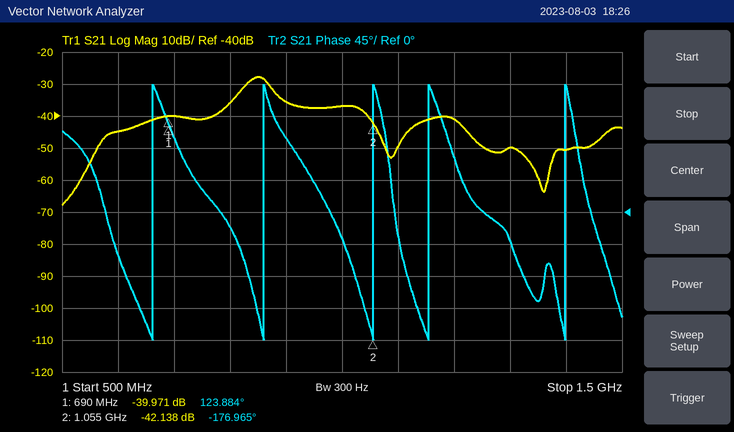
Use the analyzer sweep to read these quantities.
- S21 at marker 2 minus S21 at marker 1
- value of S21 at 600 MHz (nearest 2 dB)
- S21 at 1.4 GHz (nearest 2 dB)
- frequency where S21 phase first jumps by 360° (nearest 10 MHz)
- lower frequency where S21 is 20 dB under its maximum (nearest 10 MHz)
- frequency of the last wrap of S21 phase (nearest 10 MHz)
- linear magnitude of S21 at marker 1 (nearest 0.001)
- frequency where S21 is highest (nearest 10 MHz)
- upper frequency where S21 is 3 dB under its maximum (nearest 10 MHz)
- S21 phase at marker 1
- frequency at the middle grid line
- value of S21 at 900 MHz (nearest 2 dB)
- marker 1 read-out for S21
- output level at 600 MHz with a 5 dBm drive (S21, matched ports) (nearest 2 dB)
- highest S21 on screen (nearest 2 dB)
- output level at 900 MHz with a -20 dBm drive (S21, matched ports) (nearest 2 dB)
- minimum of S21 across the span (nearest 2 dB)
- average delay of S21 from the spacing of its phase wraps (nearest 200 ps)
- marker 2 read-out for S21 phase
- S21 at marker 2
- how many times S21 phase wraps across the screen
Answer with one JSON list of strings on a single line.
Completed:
["-2.167 dB", "-44 dB", "-50 dB", "660 MHz", "570 MHz", "1.40 GHz", "0.010", "850 MHz", "870 MHz", "123.884°", "1 GHz", "-36 dB", "-39.971 dB", "-40 dBm", "-28 dB", "-56 dBm", "-68 dB", "5.4 ns", "-176.965°", "-42.138 dB", "5"]
